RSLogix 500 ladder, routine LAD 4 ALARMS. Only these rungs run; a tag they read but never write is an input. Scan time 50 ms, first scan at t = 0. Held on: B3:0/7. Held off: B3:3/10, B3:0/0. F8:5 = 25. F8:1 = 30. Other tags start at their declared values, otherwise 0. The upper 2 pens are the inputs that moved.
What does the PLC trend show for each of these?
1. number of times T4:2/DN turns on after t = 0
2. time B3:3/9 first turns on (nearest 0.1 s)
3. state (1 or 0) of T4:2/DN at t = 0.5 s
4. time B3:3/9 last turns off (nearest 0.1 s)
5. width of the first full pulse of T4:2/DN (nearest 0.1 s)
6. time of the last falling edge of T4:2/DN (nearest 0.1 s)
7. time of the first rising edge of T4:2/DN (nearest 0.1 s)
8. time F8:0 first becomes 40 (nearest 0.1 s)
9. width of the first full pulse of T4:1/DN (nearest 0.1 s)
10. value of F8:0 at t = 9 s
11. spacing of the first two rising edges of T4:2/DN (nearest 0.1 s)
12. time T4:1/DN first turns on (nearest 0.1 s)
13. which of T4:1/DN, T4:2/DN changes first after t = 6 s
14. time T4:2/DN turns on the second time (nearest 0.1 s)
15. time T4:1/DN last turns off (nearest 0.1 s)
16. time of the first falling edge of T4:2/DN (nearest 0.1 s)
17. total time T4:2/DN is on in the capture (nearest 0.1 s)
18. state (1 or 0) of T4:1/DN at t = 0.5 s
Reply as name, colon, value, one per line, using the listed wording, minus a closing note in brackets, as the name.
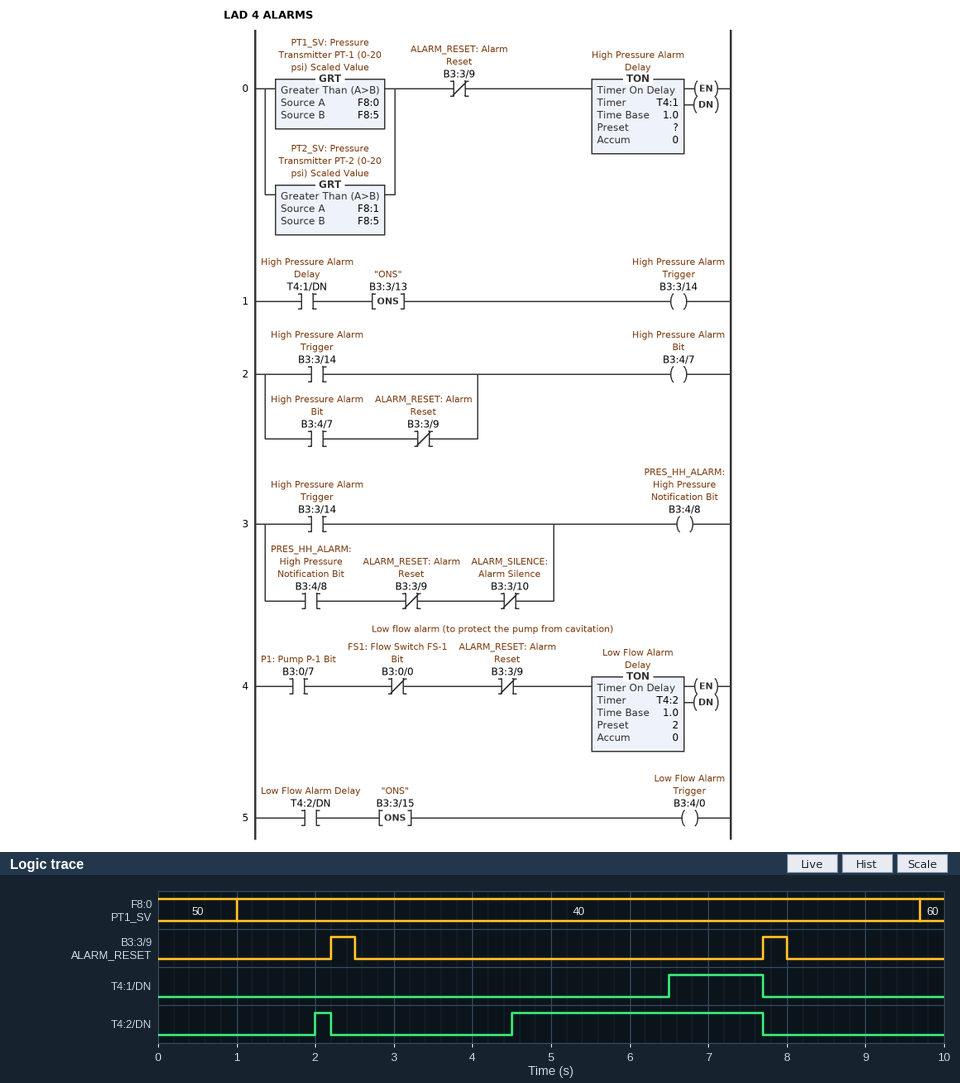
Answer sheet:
number of times T4:2/DN turns on after t = 0: 2
time B3:3/9 first turns on: 2.2 s
state (1 or 0) of T4:2/DN at t = 0.5 s: 0
time B3:3/9 last turns off: 8.0 s
width of the first full pulse of T4:2/DN: 0.2 s
time of the last falling edge of T4:2/DN: 7.7 s
time of the first rising edge of T4:2/DN: 2.0 s
time F8:0 first becomes 40: 1.0 s
width of the first full pulse of T4:1/DN: 1.2 s
value of F8:0 at t = 9 s: 40
spacing of the first two rising edges of T4:2/DN: 2.5 s
time T4:1/DN first turns on: 6.5 s
which of T4:1/DN, T4:2/DN changes first after t = 6 s: T4:1/DN
time T4:2/DN turns on the second time: 4.5 s
time T4:1/DN last turns off: 7.7 s
time of the first falling edge of T4:2/DN: 2.2 s
total time T4:2/DN is on in the capture: 3.4 s
state (1 or 0) of T4:1/DN at t = 0.5 s: 0
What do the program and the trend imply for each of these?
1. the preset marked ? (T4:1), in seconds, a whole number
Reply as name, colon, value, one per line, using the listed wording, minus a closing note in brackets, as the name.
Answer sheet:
the preset marked ? (T4:1), in seconds, a whole number: 4 s
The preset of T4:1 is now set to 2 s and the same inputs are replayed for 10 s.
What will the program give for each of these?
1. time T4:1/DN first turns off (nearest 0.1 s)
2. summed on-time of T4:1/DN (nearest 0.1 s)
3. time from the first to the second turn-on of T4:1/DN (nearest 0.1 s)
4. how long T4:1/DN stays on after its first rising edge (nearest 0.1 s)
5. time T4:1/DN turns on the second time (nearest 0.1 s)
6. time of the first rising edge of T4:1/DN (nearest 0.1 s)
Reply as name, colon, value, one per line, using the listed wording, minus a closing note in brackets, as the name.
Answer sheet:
time T4:1/DN first turns off: 2.2 s
summed on-time of T4:1/DN: 3.4 s
time from the first to the second turn-on of T4:1/DN: 2.5 s
how long T4:1/DN stays on after its first rising edge: 0.2 s
time T4:1/DN turns on the second time: 4.5 s
time of the first rising edge of T4:1/DN: 2.0 s
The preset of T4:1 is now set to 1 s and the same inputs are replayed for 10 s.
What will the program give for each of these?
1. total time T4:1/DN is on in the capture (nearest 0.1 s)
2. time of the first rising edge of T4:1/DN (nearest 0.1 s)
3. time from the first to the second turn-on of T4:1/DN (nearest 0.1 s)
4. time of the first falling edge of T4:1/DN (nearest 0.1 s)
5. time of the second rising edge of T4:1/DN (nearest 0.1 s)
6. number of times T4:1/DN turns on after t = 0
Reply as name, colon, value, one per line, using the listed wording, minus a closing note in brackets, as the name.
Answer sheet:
total time T4:1/DN is on in the capture: 6.4 s
time of the first rising edge of T4:1/DN: 1.0 s
time from the first to the second turn-on of T4:1/DN: 2.5 s
time of the first falling edge of T4:1/DN: 2.2 s
time of the second rising edge of T4:1/DN: 3.5 s
number of times T4:1/DN turns on after t = 0: 3
